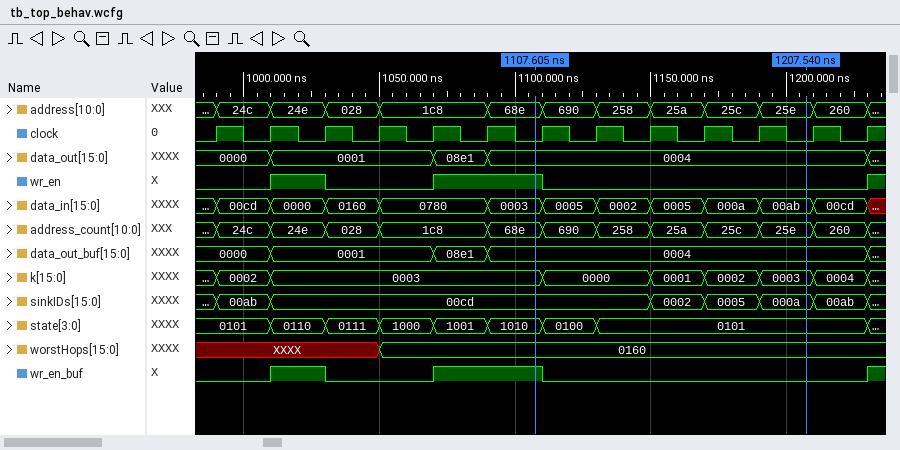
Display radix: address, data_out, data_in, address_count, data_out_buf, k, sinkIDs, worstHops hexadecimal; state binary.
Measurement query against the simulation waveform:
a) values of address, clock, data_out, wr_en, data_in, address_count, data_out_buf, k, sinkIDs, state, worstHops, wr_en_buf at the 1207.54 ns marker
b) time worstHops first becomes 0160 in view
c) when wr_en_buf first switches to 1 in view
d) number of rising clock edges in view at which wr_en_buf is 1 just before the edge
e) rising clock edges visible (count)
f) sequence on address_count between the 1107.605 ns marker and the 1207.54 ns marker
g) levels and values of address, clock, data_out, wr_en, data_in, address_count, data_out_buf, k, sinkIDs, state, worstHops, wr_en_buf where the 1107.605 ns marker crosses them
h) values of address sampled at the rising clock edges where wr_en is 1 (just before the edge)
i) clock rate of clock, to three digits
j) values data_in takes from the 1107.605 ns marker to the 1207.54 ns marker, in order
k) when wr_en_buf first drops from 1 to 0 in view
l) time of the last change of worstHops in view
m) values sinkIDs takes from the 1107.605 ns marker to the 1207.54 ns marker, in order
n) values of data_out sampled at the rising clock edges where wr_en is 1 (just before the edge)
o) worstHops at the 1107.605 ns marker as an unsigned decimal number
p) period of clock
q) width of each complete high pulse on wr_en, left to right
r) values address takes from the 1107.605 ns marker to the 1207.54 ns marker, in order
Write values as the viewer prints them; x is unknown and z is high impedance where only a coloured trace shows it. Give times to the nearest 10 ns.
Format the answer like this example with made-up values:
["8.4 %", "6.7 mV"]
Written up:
["address=25e, clock=0, data_out=0004, wr_en=0, data_in=00ab, address_count=25e, data_out_buf=0004, k=0003, sinkIDs=000a, state=0101, worstHops=0160, wr_en_buf=0", "1050 ns", "1010 ns", "3", "13", "68e, 690, 258, 25a, 25c, 25e", "address=68e, clock=0, data_out=0004, wr_en=1, data_in=0003, address_count=68e, data_out_buf=0004, k=0003, sinkIDs=00cd, state=1010, worstHops=0160, wr_en_buf=1", "24e, 1c8, 68e", "50.0 MHz", "0003, 0005, 0002, 0005, 000a, 00ab", "1030 ns", "1050 ns", "00cd, 0002, 0005, 000a", "0001, 08e1, 0004", "352", "20 ns", "20 ns, 40 ns", "68e, 690, 258, 25a, 25c, 25e"]
